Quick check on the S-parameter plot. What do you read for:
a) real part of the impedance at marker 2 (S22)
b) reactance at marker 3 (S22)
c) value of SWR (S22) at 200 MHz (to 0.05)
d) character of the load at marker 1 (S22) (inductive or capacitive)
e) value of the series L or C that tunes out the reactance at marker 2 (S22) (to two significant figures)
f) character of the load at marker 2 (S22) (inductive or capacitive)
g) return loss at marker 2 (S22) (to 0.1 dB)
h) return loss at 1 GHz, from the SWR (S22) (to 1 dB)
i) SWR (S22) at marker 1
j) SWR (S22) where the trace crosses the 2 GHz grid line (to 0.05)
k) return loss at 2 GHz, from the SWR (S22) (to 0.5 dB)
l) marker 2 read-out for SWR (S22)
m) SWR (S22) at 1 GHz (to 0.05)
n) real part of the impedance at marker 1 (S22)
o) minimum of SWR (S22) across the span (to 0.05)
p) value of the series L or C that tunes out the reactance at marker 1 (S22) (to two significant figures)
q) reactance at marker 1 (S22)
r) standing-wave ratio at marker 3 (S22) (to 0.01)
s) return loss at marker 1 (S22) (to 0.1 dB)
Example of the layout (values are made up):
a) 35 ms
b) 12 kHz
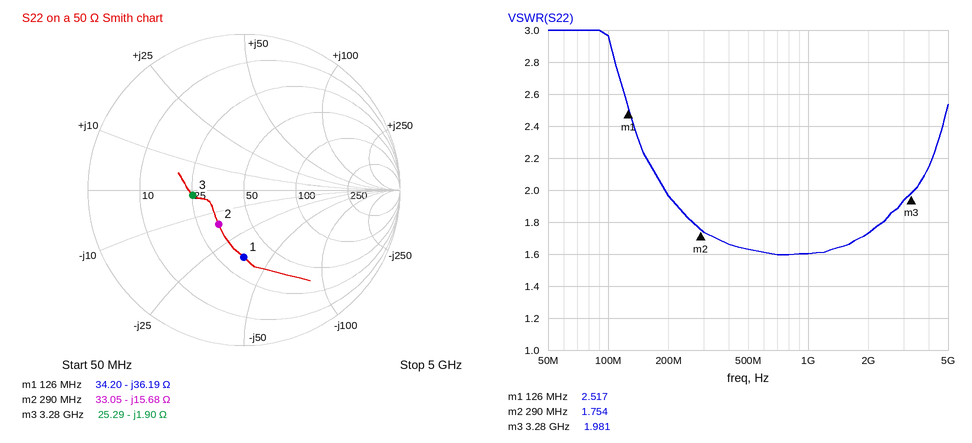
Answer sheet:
a) 33.05 Ω
b) -1.90 Ω
c) 1.95
d) capacitive
e) 8.6 nH
f) capacitive
g) 11.3 dB
h) 13 dB
i) 2.517
j) 1.75
k) 11.5 dB
l) 1.754
m) 1.60
n) 34.20 Ω
o) 1.60
p) 46 nH
q) -36.19 Ω
r) 1.98
s) 7.3 dB
